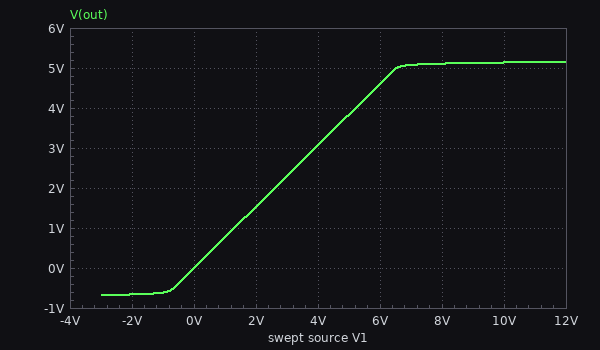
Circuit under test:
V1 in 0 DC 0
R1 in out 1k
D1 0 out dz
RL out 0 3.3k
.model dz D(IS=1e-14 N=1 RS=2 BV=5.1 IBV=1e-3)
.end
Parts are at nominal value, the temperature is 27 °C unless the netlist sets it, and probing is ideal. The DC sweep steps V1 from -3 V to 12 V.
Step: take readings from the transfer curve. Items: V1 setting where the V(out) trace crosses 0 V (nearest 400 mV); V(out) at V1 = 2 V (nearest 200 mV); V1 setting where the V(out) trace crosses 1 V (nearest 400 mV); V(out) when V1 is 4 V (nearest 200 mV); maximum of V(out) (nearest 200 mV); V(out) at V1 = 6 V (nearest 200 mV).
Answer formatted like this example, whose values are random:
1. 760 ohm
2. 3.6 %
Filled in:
1. 0 V
2. 1.6 V
3. 1.2 V
4. 3.0 V
5. 5.2 V
6. 4.6 V
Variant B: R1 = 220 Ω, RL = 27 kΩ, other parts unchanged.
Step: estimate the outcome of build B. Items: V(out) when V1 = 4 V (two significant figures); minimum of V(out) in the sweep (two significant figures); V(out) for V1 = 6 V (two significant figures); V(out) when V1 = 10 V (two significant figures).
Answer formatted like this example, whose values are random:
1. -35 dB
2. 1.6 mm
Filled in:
1. 4.0 V
2. -740 mV
3. 5.1 V
4. 5.2 V
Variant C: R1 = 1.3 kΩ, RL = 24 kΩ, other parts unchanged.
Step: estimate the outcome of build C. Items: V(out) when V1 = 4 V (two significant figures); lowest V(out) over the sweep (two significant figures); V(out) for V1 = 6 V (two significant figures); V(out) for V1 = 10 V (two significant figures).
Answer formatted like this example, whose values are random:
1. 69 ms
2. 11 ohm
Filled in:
1. 3.8 V
2. -670 mV
3. 5.1 V
4. 5.1 V
